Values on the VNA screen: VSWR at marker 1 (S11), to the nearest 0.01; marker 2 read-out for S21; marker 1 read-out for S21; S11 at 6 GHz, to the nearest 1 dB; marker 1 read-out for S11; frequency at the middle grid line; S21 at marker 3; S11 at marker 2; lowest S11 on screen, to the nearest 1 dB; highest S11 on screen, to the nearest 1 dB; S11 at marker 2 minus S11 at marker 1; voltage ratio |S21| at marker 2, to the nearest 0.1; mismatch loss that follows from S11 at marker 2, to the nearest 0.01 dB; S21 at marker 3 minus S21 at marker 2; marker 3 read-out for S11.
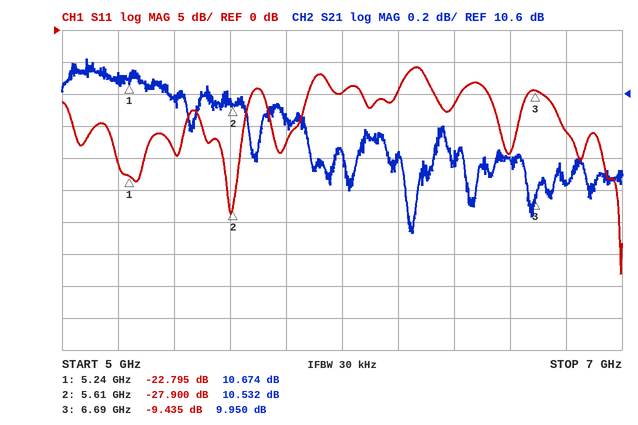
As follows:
1.16
10.532 dB
10.674 dB
-10 dB
-22.795 dB
6 GHz
9.950 dB
-27.900 dB
-38 dB
-6 dB
-5.105 dB
3.4
0.01 dB
-0.582 dB
-9.435 dB
